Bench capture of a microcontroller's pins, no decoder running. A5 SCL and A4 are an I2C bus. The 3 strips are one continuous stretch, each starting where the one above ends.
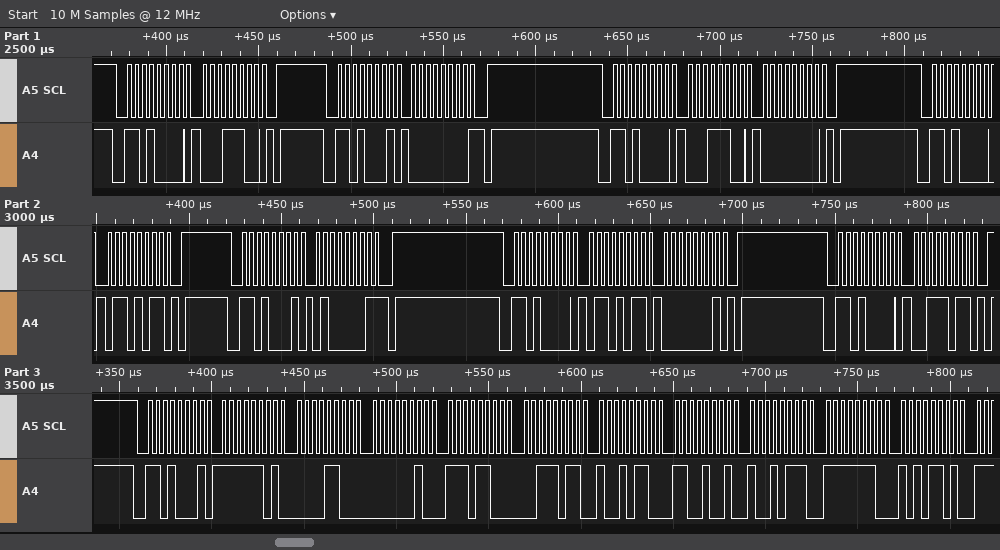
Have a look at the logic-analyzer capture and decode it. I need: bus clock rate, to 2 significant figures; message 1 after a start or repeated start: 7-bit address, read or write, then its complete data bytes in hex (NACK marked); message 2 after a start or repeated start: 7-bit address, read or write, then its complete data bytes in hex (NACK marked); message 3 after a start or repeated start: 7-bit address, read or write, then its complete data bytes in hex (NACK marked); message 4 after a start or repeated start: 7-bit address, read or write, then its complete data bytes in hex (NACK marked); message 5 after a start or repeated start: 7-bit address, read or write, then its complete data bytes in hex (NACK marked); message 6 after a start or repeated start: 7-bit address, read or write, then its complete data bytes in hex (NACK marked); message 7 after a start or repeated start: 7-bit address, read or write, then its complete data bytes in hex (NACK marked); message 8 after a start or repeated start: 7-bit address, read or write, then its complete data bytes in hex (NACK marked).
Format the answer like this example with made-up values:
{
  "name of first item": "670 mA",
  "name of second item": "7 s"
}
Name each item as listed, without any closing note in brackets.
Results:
{
  "bus clock rate, to 2 significant figures": "250 kHz",
  "message 1 after a start or repeated start: 7-bit address, read or write, then its complete data bytes in hex": "0x68 write: 1C",
  "message 2 after a start or repeated start: 7-bit address, read or write, then its complete data bytes in hex": "0x68 read: 00 NACK",
  "message 3 after a start or repeated start: 7-bit address, read or write, then its complete data bytes in hex": "0x68 write: 1C 00",
  "message 4 after a start or repeated start: 7-bit address, read or write, then its complete data bytes in hex": "0x68 write: 6B",
  "message 5 after a start or repeated start: 7-bit address, read or write, then its complete data bytes in hex": "0x68 read: 41 NACK",
  "message 6 after a start or repeated start: 7-bit address, read or write, then its complete data bytes in hex": "0x68 write: 6B 01",
  "message 7 after a start or repeated start: 7-bit address, read or write, then its complete data bytes in hex": "0x68 write: 3B",
  "message 8 after a start or repeated start: 7-bit address, read or write, then its complete data bytes in hex": "0x68 read: FD 0C 02 EC 3B 96 C9 97 FE AD"
}
